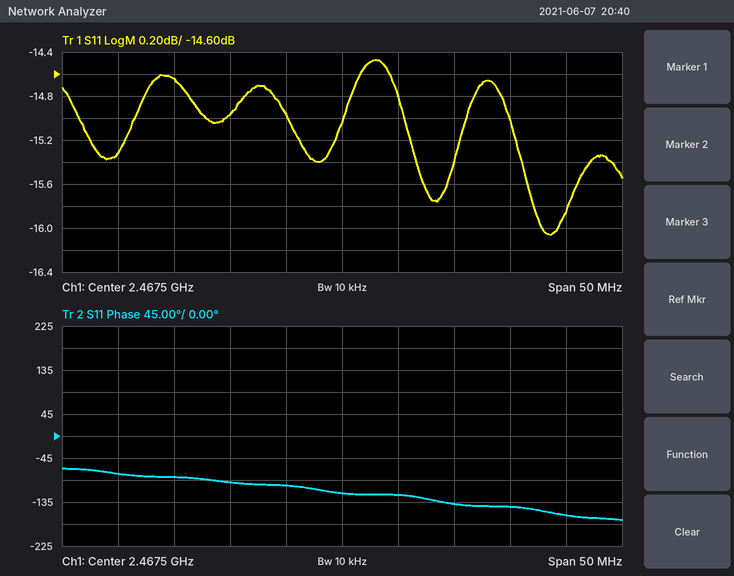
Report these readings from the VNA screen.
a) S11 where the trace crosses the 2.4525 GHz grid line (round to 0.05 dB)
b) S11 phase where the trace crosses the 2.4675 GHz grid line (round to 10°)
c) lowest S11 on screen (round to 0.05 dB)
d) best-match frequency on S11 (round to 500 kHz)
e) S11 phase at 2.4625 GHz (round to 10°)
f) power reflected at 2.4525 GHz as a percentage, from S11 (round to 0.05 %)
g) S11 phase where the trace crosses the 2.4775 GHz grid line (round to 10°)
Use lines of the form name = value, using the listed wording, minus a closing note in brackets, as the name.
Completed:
S11 where the trace crosses the 2.4525 GHz grid line = -14.65 dB
S11 phase where the trace crosses the 2.4675 GHz grid line = -120°
lowest S11 on screen = -16.05 dB
best-match frequency on S11 = 2.4860 GHz
S11 phase at 2.4625 GHz = -100°
power reflected at 2.4525 GHz as a percentage, from S11 = 3.45 %
S11 phase where the trace crosses the 2.4775 GHz grid line = -140°
